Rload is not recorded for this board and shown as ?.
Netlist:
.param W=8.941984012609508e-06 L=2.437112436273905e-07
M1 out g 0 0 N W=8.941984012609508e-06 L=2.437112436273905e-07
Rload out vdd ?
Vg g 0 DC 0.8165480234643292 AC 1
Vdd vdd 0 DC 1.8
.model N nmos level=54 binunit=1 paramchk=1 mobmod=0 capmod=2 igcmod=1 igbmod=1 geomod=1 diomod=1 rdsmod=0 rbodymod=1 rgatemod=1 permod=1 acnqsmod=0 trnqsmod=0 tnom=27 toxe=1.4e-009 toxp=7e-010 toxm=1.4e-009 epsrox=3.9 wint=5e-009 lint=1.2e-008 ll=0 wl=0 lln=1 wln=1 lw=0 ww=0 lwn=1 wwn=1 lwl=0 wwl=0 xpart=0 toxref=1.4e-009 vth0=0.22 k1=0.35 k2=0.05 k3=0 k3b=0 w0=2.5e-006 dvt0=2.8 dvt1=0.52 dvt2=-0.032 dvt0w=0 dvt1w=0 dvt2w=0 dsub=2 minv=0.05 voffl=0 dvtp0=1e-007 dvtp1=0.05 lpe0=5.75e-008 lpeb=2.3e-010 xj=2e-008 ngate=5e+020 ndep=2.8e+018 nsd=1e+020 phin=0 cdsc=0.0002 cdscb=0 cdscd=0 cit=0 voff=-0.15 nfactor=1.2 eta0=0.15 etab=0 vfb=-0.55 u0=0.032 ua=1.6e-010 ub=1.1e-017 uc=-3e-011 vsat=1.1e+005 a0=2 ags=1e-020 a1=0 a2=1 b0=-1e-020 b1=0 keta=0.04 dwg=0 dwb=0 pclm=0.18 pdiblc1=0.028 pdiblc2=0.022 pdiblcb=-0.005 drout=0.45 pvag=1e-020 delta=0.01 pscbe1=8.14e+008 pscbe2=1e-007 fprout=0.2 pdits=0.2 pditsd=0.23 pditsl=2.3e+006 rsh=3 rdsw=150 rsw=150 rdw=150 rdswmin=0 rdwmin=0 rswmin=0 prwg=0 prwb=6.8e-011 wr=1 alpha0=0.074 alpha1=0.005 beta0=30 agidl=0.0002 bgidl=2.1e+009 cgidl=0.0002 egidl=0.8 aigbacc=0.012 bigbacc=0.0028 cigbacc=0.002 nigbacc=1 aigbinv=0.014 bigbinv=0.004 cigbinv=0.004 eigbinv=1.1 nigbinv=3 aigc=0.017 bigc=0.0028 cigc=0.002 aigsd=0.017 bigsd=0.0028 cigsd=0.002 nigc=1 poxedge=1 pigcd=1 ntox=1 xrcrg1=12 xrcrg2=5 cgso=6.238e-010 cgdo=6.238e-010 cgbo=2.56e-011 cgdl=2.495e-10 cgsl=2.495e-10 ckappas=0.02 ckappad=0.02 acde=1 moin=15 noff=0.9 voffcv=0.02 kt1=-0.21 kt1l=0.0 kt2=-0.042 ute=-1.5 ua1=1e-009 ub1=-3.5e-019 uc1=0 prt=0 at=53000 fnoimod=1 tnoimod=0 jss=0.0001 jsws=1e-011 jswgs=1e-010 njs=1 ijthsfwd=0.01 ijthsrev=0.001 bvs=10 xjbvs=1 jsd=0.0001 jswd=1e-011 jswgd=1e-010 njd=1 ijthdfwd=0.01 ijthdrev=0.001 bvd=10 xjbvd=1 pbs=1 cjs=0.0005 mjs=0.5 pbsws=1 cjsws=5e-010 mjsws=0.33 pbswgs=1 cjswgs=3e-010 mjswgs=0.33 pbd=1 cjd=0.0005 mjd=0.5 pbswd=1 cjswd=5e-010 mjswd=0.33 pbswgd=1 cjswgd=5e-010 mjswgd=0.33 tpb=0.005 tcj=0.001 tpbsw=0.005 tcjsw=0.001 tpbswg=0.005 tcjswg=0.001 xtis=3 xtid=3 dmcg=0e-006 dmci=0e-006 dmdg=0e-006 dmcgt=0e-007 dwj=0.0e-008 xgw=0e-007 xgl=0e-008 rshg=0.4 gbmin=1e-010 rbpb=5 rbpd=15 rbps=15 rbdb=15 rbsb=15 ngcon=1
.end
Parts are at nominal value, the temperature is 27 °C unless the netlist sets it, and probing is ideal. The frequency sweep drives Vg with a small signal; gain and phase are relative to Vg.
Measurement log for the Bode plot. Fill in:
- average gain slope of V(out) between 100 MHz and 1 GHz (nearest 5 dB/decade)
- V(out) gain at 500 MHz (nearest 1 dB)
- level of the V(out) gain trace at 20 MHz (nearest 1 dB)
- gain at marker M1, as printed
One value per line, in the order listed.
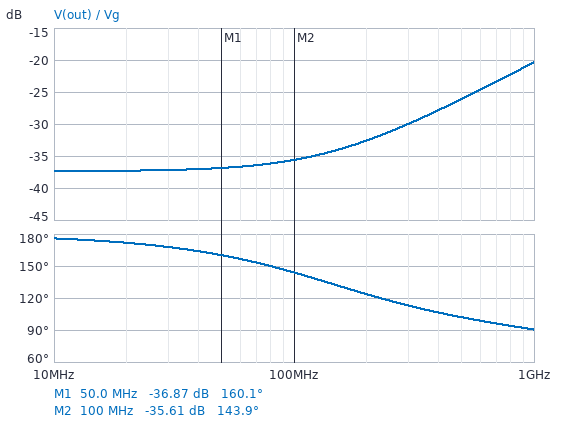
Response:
15 dB/decade
-26 dB
-37 dB
-36.87 dB
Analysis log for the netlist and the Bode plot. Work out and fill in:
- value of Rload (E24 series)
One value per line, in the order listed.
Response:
24 kΩ
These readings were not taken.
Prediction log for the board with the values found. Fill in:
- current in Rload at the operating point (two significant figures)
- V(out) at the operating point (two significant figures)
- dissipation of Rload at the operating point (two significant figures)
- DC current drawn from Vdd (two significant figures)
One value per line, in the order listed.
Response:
74 µA
24 mV
130 µW
74 µA
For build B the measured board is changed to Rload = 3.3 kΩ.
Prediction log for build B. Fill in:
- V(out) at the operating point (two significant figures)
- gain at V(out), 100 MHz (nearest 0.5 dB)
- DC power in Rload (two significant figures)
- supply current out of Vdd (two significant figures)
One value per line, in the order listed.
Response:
200 mV
-11.5 dB
770 µW
480 µA
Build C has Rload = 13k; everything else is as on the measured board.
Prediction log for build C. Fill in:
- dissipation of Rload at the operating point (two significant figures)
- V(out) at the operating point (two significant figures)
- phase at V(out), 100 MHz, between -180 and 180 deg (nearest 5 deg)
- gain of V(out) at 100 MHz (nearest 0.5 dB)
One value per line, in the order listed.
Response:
240 µW
45 mV
160 deg
-30.5 dB
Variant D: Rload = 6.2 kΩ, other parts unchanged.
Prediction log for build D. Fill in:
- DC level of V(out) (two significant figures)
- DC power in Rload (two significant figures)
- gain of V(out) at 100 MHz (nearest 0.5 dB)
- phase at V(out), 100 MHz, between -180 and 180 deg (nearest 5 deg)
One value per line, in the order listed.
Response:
98 mV
470 µW
-22.0 dB
170 deg
